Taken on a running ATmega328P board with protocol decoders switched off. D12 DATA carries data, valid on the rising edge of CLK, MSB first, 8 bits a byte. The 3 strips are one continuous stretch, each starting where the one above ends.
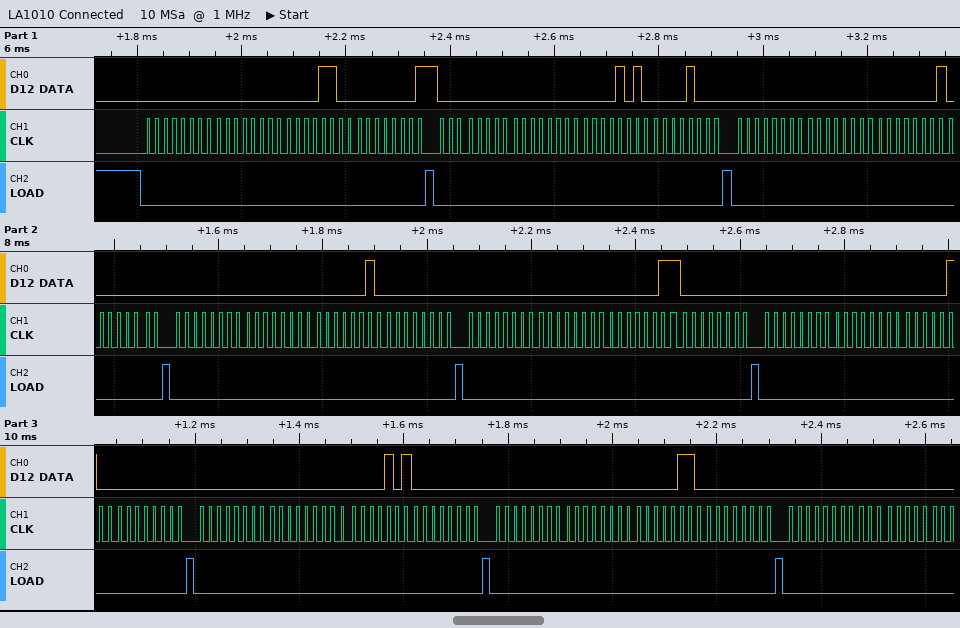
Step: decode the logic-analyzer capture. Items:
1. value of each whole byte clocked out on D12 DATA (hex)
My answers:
0x00 0x00 0x0C 0x01 0x00 0x00 0x0A 0x08 0x00 0x00 0x01 0x00 0x00 0x00 0x02 0x00 0x00 0x00 0x03 0x00 0x00 0x00 0x04 0x00 0x00 0x00 0x05 0x00 0x00 0x00 0x06 0x00 0x00 0x00
